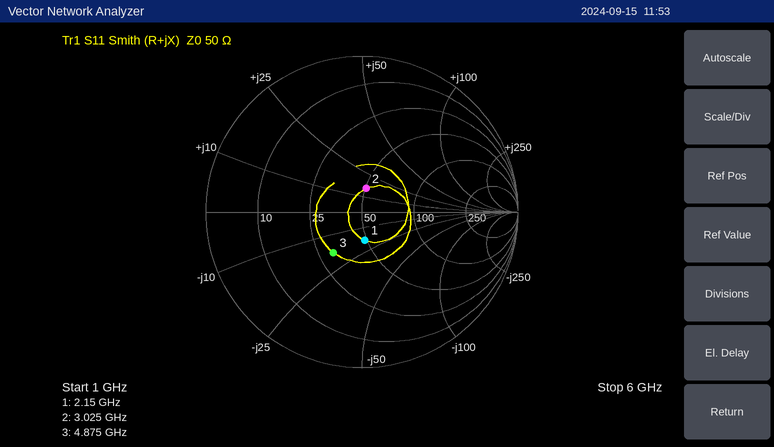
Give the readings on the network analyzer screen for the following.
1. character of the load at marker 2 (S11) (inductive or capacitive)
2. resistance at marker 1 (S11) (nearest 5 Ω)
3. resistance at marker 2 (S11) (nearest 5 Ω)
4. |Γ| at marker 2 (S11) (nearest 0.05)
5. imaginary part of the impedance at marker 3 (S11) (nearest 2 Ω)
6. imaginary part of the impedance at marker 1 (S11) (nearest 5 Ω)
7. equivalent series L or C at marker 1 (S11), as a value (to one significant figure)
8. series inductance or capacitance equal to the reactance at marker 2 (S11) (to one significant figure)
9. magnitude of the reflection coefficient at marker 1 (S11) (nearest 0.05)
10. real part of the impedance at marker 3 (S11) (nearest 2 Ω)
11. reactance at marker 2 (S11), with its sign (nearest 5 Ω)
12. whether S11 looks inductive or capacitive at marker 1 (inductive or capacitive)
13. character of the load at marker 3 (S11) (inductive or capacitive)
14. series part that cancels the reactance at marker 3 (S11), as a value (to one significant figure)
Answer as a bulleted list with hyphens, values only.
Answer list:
- inductive
- 50 Ω
- 50 Ω
- 0.15
- -18 Ω
- -20 Ω
- 4 pF
- 800 pH
- 0.20
- 30 Ω
- +15 Ω
- capacitive
- capacitive
- 600 pH
